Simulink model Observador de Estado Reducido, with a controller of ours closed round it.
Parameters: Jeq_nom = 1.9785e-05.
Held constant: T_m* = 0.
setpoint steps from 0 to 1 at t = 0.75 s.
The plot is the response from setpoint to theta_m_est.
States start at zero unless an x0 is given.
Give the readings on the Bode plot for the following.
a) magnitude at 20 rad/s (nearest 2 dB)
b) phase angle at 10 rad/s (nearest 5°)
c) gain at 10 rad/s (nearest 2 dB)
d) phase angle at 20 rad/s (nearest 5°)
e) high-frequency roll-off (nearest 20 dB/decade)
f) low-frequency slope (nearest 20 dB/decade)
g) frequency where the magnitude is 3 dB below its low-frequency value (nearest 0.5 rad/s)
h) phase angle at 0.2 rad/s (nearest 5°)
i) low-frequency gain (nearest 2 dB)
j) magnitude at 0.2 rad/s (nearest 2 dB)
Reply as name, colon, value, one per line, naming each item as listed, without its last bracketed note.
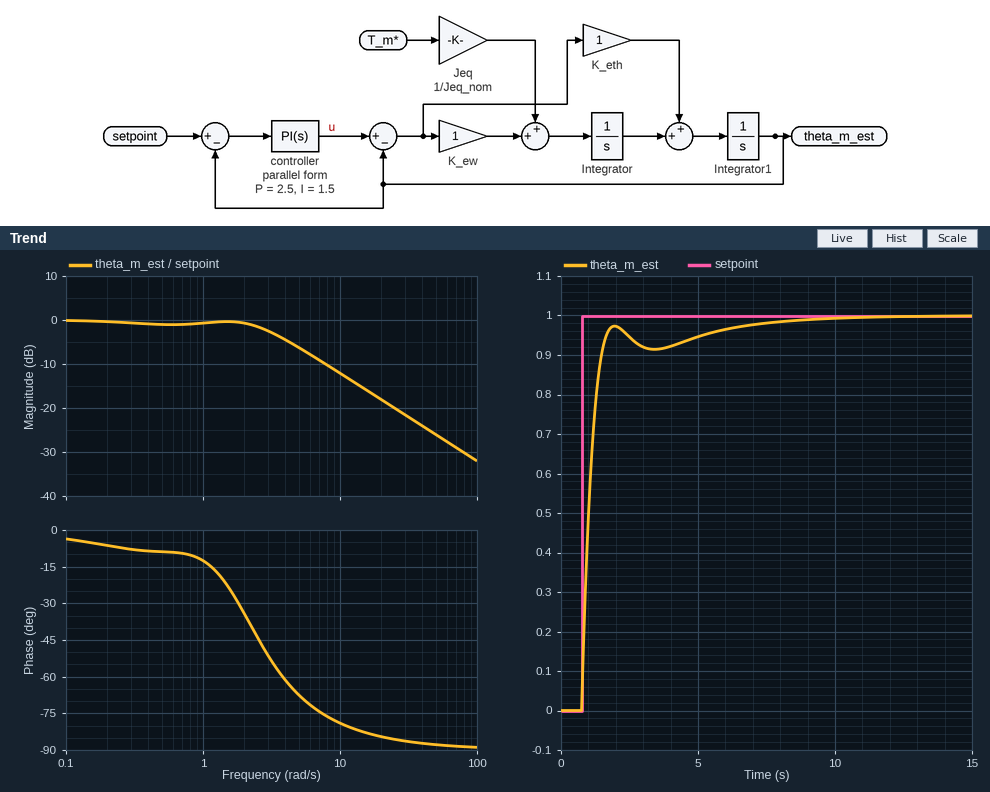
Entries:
magnitude at 20 rad/s: -18 dB
phase angle at 10 rad/s: -80°
gain at 10 rad/s: -12 dB
phase angle at 20 rad/s: -85°
high-frequency roll-off: -20 dB/decade
low-frequency slope: 0 dB/decade
frequency where the magnitude is 3 dB below its low-frequency value: 3.5 rad/s
phase angle at 0.2 rad/s: -5°
low-frequency gain: 0 dB
magnitude at 0.2 rad/s: 0 dB
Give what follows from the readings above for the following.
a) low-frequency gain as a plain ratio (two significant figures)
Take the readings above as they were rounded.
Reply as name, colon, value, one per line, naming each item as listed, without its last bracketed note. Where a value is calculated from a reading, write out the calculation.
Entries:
low-frequency gain as a plain ratio: 10^(0 / 20) = 1.0
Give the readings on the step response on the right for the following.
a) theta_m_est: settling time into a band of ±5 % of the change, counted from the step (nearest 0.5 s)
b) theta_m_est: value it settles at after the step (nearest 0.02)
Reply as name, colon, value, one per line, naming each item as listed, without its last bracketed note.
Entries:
theta_m_est: settling time into a band of ±5 % of the change, counted from the step: 4.5 s
theta_m_est: value it settles at after the step: 1.00
